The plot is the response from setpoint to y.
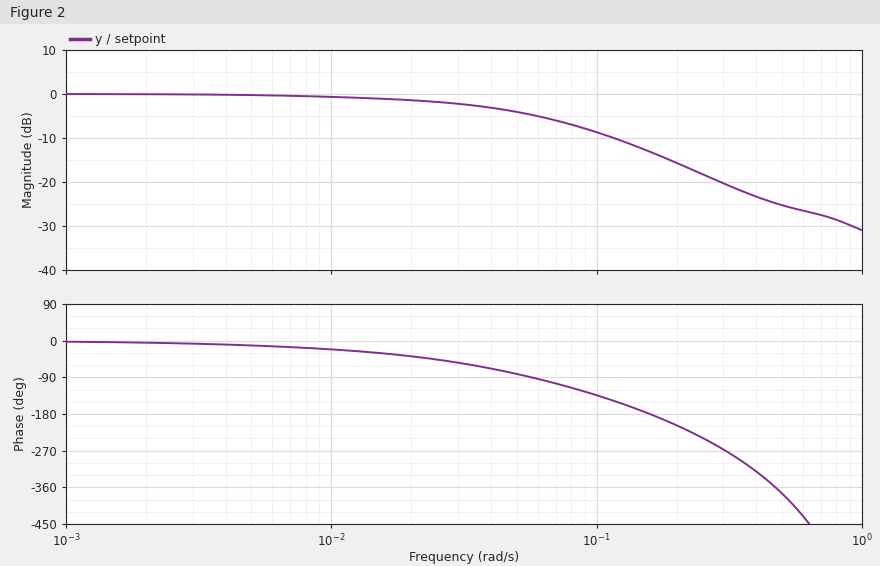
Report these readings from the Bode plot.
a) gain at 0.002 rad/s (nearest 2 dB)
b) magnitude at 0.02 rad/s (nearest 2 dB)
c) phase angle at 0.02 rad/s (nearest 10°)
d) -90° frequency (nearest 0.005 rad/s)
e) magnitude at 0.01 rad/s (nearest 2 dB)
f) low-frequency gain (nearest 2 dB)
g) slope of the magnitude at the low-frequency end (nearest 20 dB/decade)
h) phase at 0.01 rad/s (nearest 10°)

0 dB
-2 dB
-40°
0.055 rad/s
0 dB
0 dB
0 dB/decade
-20°
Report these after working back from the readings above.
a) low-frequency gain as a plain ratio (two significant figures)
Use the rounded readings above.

1.0
